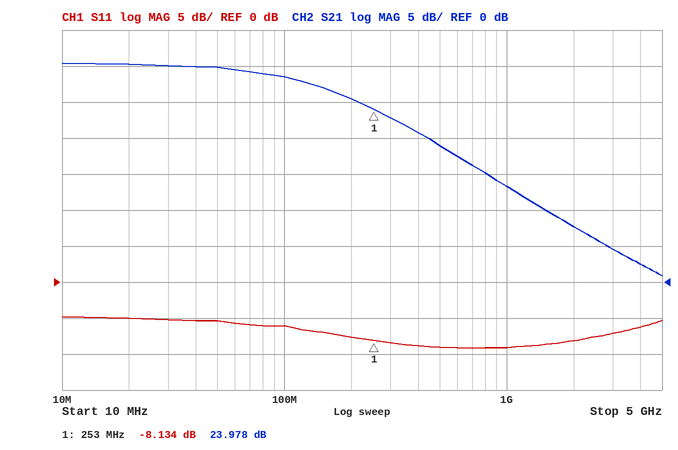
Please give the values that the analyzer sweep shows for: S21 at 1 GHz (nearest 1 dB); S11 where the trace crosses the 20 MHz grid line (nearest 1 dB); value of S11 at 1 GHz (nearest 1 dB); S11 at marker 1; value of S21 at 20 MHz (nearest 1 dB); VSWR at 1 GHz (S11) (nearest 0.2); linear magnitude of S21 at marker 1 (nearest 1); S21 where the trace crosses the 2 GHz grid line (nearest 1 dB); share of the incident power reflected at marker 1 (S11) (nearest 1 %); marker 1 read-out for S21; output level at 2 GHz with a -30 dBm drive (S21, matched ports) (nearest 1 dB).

13 dB
-5 dB
-9 dB
-8.134 dB
30 dB
2.0
16
8 dB
15 %
23.978 dB
-22 dBm
